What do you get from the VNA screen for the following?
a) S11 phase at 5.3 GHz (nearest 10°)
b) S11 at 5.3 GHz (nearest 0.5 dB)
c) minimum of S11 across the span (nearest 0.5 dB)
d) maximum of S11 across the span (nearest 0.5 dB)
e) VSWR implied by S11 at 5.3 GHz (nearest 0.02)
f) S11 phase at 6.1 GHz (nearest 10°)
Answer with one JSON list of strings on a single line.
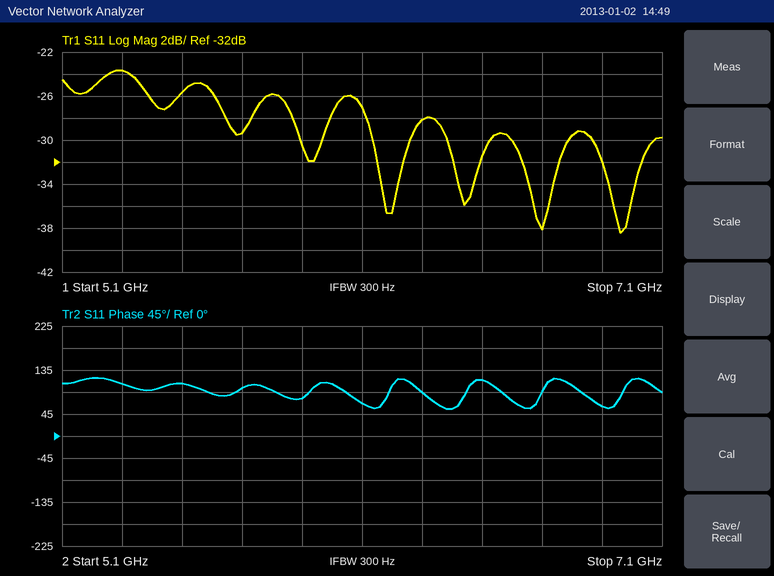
["110°", "-23.5 dB", "-38.5 dB", "-23.5 dB", "1.14", "70°"]
